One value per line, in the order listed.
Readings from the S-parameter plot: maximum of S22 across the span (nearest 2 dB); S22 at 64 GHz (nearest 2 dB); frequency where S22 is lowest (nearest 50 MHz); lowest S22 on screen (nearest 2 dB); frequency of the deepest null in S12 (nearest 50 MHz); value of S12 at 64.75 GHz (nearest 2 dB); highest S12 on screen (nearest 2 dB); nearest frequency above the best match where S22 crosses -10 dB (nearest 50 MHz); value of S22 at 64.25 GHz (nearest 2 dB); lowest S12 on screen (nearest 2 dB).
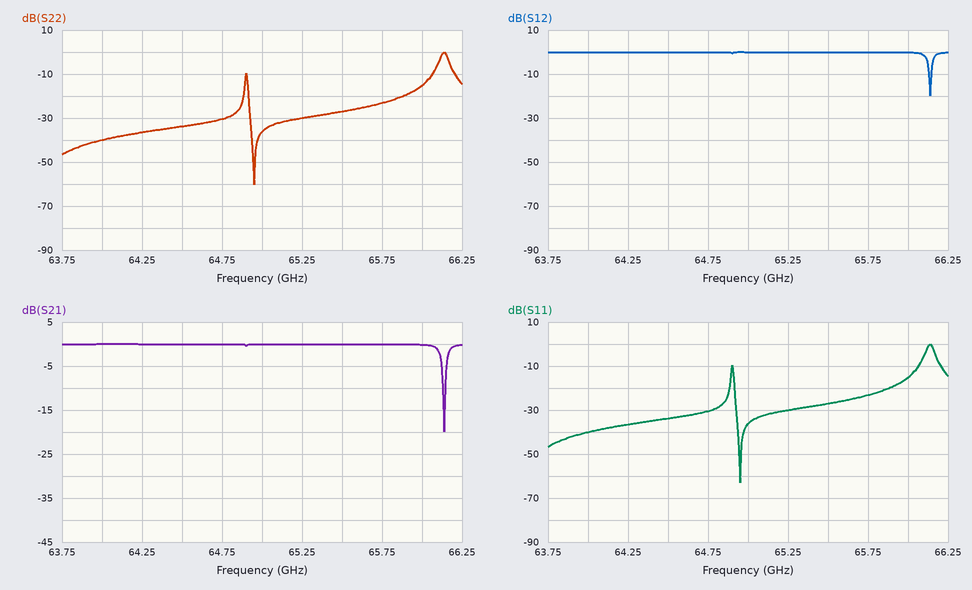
0 dB
-40 dB
64.95 GHz
-60 dB
66.15 GHz
0 dB
0 dB
66.05 GHz
-36 dB
-20 dB
